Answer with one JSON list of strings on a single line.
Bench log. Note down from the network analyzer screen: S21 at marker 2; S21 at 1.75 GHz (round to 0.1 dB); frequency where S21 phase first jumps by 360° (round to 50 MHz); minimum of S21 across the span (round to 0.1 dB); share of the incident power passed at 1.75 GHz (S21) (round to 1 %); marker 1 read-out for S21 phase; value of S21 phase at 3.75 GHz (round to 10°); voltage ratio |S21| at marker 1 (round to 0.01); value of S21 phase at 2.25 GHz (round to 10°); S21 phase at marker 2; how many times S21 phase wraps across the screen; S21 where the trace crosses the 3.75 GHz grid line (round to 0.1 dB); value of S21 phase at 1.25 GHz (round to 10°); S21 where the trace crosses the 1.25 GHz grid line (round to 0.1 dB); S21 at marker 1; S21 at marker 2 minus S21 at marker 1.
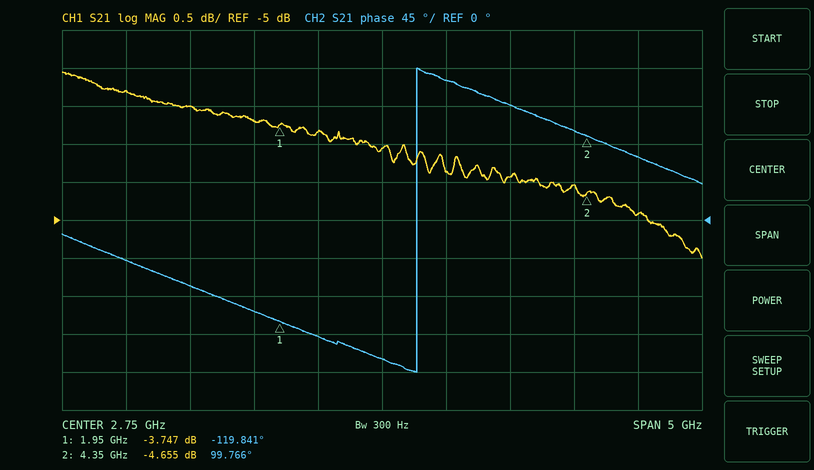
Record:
["-4.655 dB", "-3.7 dB", "3.00 GHz", "-5.5 dB", "43 %", "-119.841°", "140°", "0.65", "-140°", "99.766°", "1", "-4.4 dB", "-80°", "-3.5 dB", "-3.747 dB", "-0.908 dB"]
